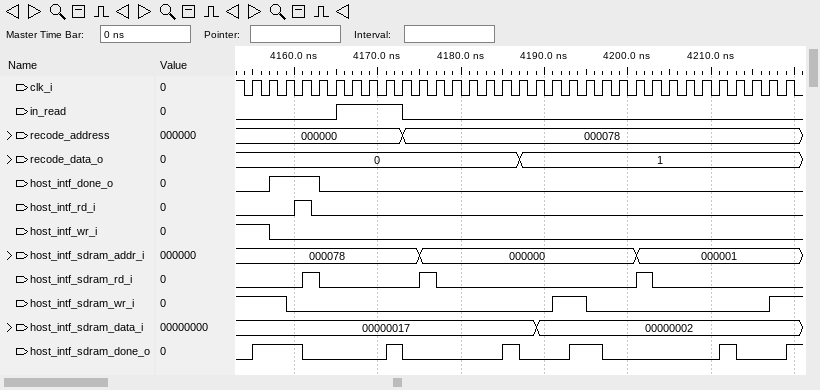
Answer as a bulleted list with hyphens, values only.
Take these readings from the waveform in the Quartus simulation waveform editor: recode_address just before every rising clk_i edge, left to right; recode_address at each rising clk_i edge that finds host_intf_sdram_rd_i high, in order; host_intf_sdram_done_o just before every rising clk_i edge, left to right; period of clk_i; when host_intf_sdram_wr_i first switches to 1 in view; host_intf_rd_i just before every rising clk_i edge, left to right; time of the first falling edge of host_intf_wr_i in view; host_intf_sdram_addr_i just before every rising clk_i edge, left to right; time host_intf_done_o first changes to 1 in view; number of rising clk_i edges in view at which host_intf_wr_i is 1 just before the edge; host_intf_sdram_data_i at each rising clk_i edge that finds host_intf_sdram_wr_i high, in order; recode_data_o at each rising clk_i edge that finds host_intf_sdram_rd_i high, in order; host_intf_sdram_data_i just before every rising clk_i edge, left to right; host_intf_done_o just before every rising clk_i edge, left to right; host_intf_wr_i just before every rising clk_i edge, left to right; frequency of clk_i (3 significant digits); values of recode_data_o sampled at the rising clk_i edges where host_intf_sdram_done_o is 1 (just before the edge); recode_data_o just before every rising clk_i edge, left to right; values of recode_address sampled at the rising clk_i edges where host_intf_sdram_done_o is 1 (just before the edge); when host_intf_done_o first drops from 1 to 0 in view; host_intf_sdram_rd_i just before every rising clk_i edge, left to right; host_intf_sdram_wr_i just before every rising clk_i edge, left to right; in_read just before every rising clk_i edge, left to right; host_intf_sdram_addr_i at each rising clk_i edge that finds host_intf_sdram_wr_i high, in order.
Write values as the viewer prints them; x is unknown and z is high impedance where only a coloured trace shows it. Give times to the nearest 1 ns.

- 000000, 000000, 000000, 000000, 000000, 000000, 000000, 000000, 000000, 000000, 000078, 000078, 000078, 000078, 000078, 000078, 000078, 000078, 000078, 000078, 000078, 000078, 000078, 000078, 000078, 000078, 000078, 000078, 000078, 000078, 000078, 000078, 000078
- 000000, 000078, 000078
- 0 1 1 1 0 0 0 0 0 1 0 0 0 0 0 0 1 0 0 0 1 1 0 0 0 0 0 0 0 1 0 0 0
- 2 ns
- 4191 ns
- 0 0 0 1 0 0 0 0 0 0 0 0 0 0 0 0 0 0 0 0 0 0 0 0 0 0 0 0 0 0 0 0 0
- 4157 ns
- 000078, 000078, 000078, 000078, 000078, 000078, 000078, 000078, 000078, 000078, 000078, 000000, 000000, 000000, 000000, 000000, 000000, 000000, 000000, 000000, 000000, 000000, 000000, 000000, 000001, 000001, 000001, 000001, 000001, 000001, 000001, 000001, 000001
- 4157 ns
- 2
- 00000017, 00000017, 00000017, 00000002, 00000002, 00000002
- 0, 0, 1
- 00000017, 00000017, 00000017, 00000017, 00000017, 00000017, 00000017, 00000017, 00000017, 00000017, 00000017, 00000017, 00000017, 00000017, 00000017, 00000017, 00000017, 00000017, 00000002, 00000002, 00000002, 00000002, 00000002, 00000002, 00000002, 00000002, 00000002, 00000002, 00000002, 00000002, 00000002, 00000002, 00000002
- 0 0 1 1 1 0 0 0 0 0 0 0 0 0 0 0 0 0 0 0 0 0 0 0 0 0 0 0 0 0 0 0 0
- 1 1 0 0 0 0 0 0 0 0 0 0 0 0 0 0 0 0 0 0 0 0 0 0 0 0 0 0 0 0 0 0 0
- 500 MHz
- 0, 0, 0, 0, 0, 1, 1, 1
- 0, 0, 0, 0, 0, 0, 0, 0, 0, 0, 0, 0, 0, 0, 0, 0, 0, 1, 1, 1, 1, 1, 1, 1, 1, 1, 1, 1, 1, 1, 1, 1, 1
- 000000, 000000, 000000, 000000, 000078, 000078, 000078, 000078
- 4163 ns
- 0 0 0 0 1 0 0 0 0 0 0 1 0 0 0 0 0 0 0 0 0 0 0 0 1 0 0 0 0 0 0 0 0
- 1 1 1 0 0 0 0 0 0 0 0 0 0 0 0 0 0 0 0 1 1 0 0 0 0 0 0 0 0 0 0 0 1
- 0 0 0 0 0 0 1 1 1 1 0 0 0 0 0 0 0 0 0 0 0 0 0 0 0 0 0 0 0 0 0 0 0
- 000078, 000078, 000078, 000000, 000000, 000001
